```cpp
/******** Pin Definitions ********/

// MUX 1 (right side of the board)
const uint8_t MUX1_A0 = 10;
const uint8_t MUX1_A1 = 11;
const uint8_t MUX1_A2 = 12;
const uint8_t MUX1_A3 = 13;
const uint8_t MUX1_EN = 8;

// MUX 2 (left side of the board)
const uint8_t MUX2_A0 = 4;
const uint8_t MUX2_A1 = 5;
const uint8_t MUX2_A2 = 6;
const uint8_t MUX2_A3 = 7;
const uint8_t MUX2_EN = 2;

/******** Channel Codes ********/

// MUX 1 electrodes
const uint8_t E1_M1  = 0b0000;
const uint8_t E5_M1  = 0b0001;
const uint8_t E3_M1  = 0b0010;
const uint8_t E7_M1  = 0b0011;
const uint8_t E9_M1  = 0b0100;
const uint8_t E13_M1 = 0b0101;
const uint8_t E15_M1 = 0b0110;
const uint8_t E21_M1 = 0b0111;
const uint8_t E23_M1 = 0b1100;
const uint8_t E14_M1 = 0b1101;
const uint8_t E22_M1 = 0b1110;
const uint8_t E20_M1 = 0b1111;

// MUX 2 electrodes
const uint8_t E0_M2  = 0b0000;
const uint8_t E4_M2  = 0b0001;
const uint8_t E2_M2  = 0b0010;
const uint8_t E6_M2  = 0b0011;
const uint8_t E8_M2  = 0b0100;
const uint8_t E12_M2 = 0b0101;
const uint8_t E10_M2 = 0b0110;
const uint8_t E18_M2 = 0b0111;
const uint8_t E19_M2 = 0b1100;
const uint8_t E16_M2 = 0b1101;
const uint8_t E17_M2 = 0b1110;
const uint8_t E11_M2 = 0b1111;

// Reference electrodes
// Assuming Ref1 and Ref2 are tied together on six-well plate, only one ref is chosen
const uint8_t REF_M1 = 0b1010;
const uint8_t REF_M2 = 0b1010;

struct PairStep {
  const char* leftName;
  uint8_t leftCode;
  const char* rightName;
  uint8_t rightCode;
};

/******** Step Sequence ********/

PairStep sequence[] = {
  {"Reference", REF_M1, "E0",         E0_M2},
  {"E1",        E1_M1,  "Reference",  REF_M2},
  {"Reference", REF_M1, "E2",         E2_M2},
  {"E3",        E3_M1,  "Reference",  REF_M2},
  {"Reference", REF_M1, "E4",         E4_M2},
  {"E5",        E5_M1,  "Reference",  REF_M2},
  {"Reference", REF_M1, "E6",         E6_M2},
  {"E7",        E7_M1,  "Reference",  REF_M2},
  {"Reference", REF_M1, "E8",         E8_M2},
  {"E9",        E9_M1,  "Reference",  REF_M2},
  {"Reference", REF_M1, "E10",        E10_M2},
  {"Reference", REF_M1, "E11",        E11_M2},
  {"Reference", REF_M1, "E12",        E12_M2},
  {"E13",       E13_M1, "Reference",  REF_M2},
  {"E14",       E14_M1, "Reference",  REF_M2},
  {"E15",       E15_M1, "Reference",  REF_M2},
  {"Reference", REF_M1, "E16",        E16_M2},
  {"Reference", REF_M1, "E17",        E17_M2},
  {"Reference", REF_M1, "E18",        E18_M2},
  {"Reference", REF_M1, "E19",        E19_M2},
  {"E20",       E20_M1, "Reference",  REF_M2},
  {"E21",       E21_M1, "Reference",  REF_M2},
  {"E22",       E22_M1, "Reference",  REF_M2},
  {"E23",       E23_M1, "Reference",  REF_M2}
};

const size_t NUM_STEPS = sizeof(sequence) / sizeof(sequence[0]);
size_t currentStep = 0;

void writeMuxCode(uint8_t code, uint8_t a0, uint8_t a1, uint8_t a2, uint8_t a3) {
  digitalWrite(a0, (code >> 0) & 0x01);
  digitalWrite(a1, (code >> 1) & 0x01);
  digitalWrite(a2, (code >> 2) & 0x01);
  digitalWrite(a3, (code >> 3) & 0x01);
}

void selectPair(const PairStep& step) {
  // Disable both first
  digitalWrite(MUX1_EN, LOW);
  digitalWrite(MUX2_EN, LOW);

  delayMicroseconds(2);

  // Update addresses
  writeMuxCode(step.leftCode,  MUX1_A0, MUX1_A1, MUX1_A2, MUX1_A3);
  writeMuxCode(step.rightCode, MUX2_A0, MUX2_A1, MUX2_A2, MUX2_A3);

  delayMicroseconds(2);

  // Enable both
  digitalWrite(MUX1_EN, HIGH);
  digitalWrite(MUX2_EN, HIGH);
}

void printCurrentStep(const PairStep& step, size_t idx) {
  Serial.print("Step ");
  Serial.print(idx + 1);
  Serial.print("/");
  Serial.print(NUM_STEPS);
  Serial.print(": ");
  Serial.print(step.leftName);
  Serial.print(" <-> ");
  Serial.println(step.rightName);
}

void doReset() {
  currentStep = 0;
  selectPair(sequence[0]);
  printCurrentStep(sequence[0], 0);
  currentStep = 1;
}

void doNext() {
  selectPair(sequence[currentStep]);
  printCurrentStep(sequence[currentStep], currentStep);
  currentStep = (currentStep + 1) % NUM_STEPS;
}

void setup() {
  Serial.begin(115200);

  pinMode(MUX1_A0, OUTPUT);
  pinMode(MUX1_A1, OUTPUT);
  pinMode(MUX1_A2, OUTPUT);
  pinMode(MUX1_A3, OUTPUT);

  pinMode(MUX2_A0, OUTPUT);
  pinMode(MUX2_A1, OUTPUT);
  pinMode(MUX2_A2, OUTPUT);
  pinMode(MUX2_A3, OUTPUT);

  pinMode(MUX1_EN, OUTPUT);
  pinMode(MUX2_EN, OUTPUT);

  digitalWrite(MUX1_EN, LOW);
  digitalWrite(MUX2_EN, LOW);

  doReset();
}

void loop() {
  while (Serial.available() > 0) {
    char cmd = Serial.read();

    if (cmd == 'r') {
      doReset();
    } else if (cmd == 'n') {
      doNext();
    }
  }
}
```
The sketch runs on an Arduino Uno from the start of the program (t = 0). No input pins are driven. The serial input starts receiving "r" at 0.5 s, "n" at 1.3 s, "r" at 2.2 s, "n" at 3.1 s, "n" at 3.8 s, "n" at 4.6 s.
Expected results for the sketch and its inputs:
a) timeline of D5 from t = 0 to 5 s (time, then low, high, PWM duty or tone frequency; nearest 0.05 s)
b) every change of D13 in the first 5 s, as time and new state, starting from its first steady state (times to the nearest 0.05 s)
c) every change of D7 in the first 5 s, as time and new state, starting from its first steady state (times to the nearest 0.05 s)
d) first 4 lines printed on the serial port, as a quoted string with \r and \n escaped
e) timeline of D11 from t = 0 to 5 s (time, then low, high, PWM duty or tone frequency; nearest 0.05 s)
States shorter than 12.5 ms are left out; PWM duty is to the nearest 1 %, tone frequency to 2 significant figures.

0 s low; 1.3 s high; 2.2 s low; 3.1 s high
0 s high; 1.3 s low; 2.2 s high; 3.1 s low; 3.8 s high; 4.6 s low
0 s low; 1.3 s high; 2.2 s low; 3.1 s high; 3.8 s low; 4.6 s high
"Step 1/24: Reference <-> E0\r\nStep 1/24: Reference <-> E0\r\nStep 2/24: E1 <-> Reference\r\nStep 1/24: Reference <-> E0\r\n"
0 s high; 1.3 s low; 2.2 s high; 3.1 s low; 3.8 s high
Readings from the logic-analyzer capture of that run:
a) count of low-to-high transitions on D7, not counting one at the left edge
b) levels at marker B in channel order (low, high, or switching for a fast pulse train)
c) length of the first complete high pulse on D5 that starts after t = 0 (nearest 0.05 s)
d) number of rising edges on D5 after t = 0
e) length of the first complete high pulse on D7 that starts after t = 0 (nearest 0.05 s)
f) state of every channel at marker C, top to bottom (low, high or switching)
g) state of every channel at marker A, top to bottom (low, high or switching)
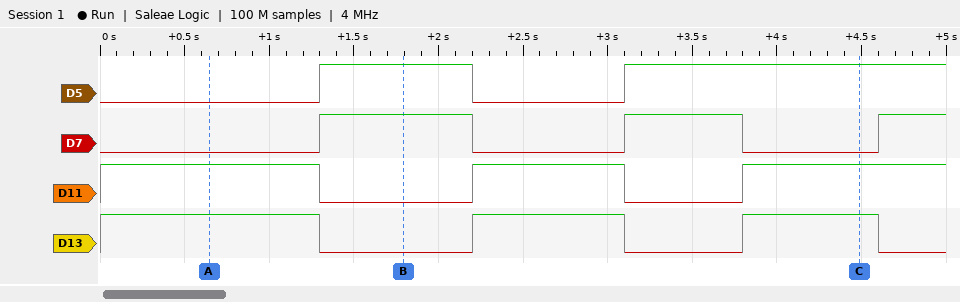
3
D5 high, D7 high, D11 low, D13 low
0.90 s
2
0.90 s
D5 high, D7 low, D11 high, D13 high
D5 low, D7 low, D11 high, D13 high
